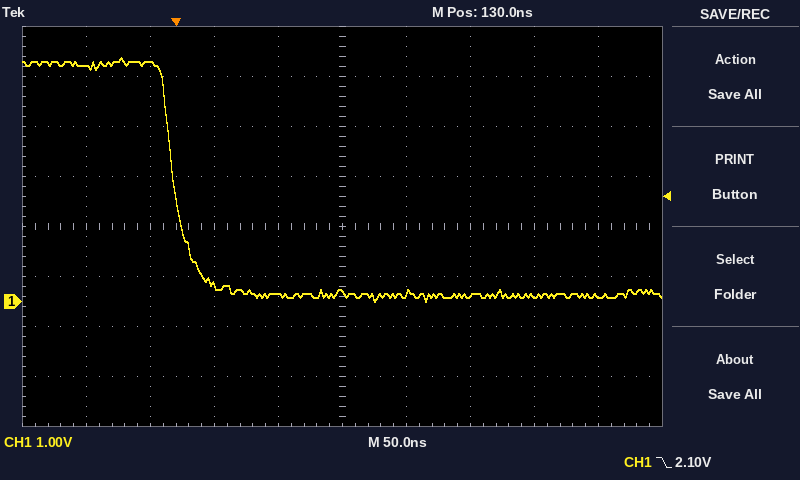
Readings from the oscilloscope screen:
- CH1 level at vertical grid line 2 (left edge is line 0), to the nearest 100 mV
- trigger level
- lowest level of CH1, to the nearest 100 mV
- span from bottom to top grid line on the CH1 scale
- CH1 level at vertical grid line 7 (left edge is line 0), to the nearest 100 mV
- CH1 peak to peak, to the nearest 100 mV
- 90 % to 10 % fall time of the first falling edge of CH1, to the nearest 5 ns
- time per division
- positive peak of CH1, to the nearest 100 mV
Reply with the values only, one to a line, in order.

4.8 V
2.10 V
0.0 V
8 V
100 mV
4.9 V
30 ns
50 ns
4.9 V
